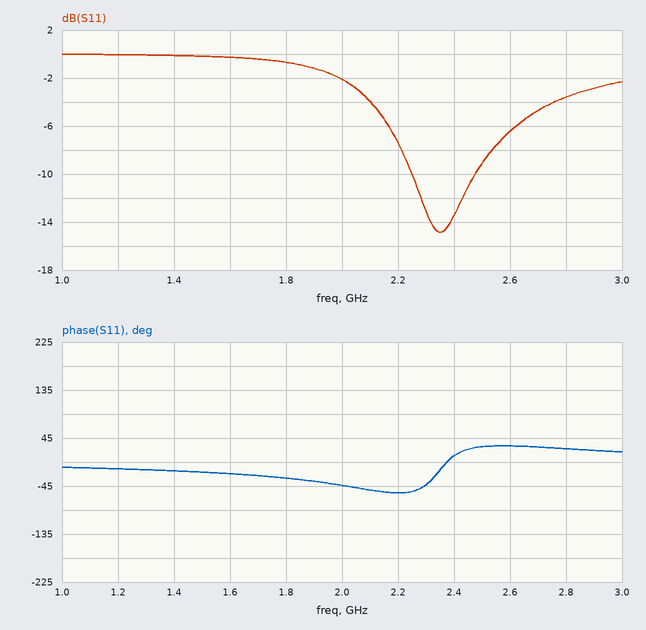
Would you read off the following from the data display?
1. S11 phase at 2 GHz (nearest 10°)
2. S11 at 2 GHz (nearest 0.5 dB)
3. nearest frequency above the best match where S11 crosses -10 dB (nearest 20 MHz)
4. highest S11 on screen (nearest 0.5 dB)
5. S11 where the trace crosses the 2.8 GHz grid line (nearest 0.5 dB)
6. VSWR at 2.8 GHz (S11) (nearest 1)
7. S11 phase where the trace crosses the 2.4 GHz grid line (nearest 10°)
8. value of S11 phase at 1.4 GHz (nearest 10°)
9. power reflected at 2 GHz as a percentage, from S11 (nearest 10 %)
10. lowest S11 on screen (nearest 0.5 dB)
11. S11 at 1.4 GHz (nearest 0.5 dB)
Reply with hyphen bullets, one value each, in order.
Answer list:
- -40°
- -2.0 dB
- 2.48 GHz
- 0.0 dB
- -3.5 dB
- 5
- 10°
- -20°
- 60 %
- -15.0 dB
- 0.0 dB
